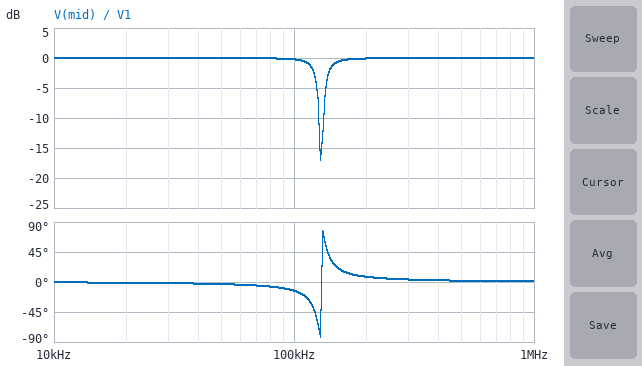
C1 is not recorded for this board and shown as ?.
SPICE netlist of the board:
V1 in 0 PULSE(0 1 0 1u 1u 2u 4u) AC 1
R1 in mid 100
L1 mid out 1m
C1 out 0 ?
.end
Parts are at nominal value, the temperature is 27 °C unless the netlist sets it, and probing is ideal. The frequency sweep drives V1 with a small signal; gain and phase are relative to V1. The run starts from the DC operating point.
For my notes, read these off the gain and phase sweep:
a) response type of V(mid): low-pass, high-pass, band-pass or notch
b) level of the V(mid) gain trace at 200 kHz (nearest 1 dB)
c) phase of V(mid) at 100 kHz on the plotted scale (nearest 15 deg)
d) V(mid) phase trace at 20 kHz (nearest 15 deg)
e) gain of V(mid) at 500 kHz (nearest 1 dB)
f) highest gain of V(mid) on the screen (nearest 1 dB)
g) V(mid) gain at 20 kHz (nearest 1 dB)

notch
0 dB
-15 deg
0 deg
0 dB
0 dB
0 dB
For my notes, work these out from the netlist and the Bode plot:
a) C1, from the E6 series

1.5 nF
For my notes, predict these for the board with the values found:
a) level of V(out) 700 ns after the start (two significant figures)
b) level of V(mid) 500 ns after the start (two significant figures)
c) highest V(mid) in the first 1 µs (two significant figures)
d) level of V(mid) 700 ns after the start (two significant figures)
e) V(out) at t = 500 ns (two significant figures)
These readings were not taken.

37 mV
490 mV
950 mV
680 mV
14 mV
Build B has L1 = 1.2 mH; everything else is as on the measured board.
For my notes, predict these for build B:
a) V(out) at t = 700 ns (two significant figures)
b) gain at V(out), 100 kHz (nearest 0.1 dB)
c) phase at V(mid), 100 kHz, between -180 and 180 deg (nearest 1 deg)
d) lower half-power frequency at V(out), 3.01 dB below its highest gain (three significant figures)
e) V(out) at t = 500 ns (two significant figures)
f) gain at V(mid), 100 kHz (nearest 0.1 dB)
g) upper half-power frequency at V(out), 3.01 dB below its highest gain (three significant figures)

31 mV
10.3 dB
-18 deg
111 kHz
11 mV
-0.4 dB
125 kHz
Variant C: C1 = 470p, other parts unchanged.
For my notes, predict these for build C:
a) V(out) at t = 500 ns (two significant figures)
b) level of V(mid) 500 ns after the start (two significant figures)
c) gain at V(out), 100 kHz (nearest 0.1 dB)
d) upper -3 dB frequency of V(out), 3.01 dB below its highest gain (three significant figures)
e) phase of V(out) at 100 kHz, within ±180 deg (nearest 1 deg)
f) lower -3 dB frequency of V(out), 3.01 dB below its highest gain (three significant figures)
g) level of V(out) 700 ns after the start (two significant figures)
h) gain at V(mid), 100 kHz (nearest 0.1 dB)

43 mV
490 mV
1.8 dB
240 kHz
-2 deg
224 kHz
110 mV
0 dB
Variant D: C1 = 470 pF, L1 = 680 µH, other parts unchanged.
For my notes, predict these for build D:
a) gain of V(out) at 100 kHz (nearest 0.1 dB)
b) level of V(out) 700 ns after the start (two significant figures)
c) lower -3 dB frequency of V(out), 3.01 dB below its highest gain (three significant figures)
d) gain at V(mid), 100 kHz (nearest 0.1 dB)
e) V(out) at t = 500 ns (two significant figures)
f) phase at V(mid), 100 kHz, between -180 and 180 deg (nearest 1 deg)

1.2 dB
160 mV
269 kHz
0 dB
62 mV
-2 deg
